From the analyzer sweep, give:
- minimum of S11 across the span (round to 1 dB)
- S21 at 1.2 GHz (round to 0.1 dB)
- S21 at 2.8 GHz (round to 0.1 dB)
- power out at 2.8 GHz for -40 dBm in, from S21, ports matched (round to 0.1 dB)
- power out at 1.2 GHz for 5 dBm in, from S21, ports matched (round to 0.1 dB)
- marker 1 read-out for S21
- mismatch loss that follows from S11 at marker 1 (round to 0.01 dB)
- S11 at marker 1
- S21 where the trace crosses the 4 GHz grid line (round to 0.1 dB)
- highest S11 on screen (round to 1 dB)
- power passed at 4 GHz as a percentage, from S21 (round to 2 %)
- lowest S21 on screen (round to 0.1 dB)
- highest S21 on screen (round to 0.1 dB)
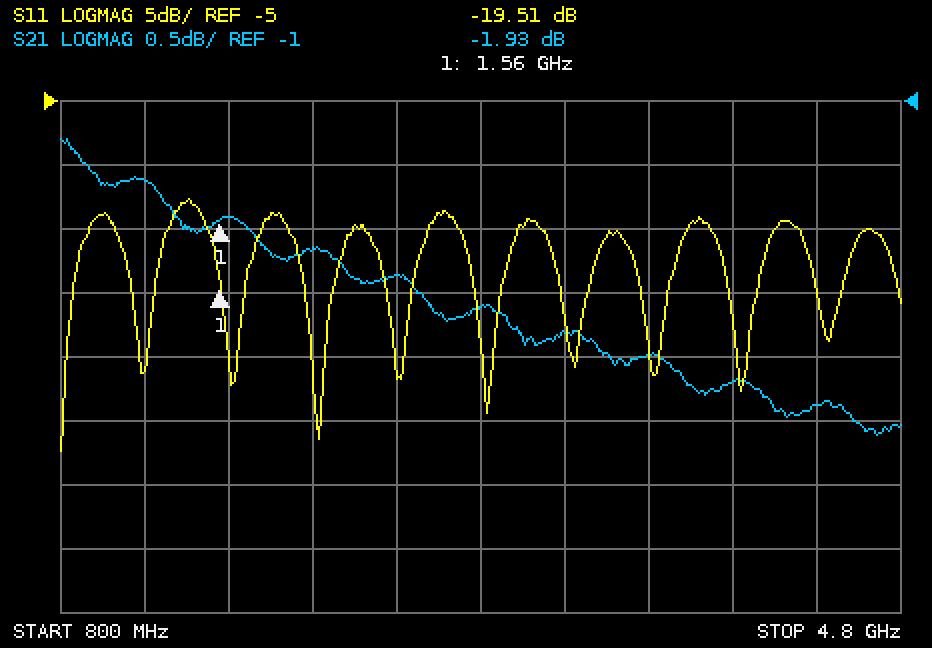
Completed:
-32 dB
-1.6 dB
-2.6 dB
-42.6 dBm
3.4 dBm
-1.93 dB
0.05 dB
-19.51 dB
-3.2 dB
-13 dB
48 %
-3.6 dB
-1.3 dB
